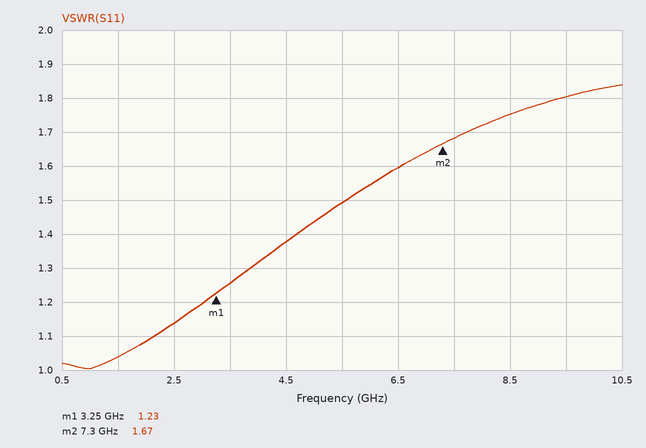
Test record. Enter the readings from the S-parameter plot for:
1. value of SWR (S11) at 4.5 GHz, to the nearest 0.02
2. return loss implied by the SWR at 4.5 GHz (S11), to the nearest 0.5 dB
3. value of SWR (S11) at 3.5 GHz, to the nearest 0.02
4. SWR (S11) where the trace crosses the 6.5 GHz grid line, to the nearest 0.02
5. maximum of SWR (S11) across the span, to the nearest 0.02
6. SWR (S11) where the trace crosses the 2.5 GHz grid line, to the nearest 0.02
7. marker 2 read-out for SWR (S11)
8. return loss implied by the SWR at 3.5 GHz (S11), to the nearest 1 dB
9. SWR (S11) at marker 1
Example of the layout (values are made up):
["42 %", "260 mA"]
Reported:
["1.38", "16.0 dB", "1.26", "1.60", "1.84", "1.14", "1.67", "19 dB", "1.23"]
